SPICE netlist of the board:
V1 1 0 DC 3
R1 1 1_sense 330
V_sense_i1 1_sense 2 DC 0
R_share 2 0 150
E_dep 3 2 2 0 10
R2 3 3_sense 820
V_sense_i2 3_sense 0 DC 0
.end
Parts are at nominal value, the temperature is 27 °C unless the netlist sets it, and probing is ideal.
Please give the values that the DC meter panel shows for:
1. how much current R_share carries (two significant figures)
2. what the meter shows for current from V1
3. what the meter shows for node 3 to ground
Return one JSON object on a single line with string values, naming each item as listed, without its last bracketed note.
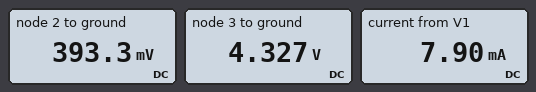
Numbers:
{"how much current R_share carries": "2.6 mA", "what the meter shows for current from V1": "7.90 mA", "what the meter shows for node 3 to ground": "4.327 V"}
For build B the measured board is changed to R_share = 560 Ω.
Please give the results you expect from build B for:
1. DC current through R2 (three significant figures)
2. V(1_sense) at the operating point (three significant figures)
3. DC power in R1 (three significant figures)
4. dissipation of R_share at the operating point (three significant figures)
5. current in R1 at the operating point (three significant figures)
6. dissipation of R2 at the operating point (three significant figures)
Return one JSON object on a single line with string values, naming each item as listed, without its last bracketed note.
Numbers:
{"DC current through R2": "6.69 mA", "V(1_sense) at the operating point": "499 mV", "DC power in R1": "19.0 mW", "dissipation of R_share at the operating point": "444 µW", "current in R1 at the operating point": "7.58 mA", "dissipation of R2 at the operating point": "36.7 mW"}
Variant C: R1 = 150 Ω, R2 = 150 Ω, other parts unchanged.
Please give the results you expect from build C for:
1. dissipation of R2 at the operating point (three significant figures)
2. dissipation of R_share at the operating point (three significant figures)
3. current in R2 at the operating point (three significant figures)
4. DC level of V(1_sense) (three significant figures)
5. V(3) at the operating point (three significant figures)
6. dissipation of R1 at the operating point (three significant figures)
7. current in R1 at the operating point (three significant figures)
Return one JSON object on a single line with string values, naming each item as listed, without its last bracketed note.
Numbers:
{"dissipation of R2 at the operating point": "43.0 mW", "dissipation of R_share at the operating point": "355 µW", "current in R2 at the operating point": "16.9 mA", "DC level of V(1_sense)": "231 mV", "V(3) at the operating point": "2.54 V", "dissipation of R1 at the operating point": "51.1 mW", "current in R1 at the operating point": "18.5 mA"}
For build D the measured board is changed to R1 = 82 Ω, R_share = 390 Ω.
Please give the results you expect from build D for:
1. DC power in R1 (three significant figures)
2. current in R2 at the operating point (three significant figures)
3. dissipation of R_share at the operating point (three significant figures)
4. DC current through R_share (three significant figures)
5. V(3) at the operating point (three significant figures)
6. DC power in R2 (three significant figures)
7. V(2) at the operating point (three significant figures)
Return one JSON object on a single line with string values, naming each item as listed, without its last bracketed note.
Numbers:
{"DC power in R1": "35.3 mW", "current in R2 at the operating point": "17.4 mA", "dissipation of R_share at the operating point": "4.32 mW", "DC current through R_share": "3.33 mA", "V(3) at the operating point": "14.3 V", "DC power in R2": "249 mW", "V(2) at the operating point": "1.30 V"}
